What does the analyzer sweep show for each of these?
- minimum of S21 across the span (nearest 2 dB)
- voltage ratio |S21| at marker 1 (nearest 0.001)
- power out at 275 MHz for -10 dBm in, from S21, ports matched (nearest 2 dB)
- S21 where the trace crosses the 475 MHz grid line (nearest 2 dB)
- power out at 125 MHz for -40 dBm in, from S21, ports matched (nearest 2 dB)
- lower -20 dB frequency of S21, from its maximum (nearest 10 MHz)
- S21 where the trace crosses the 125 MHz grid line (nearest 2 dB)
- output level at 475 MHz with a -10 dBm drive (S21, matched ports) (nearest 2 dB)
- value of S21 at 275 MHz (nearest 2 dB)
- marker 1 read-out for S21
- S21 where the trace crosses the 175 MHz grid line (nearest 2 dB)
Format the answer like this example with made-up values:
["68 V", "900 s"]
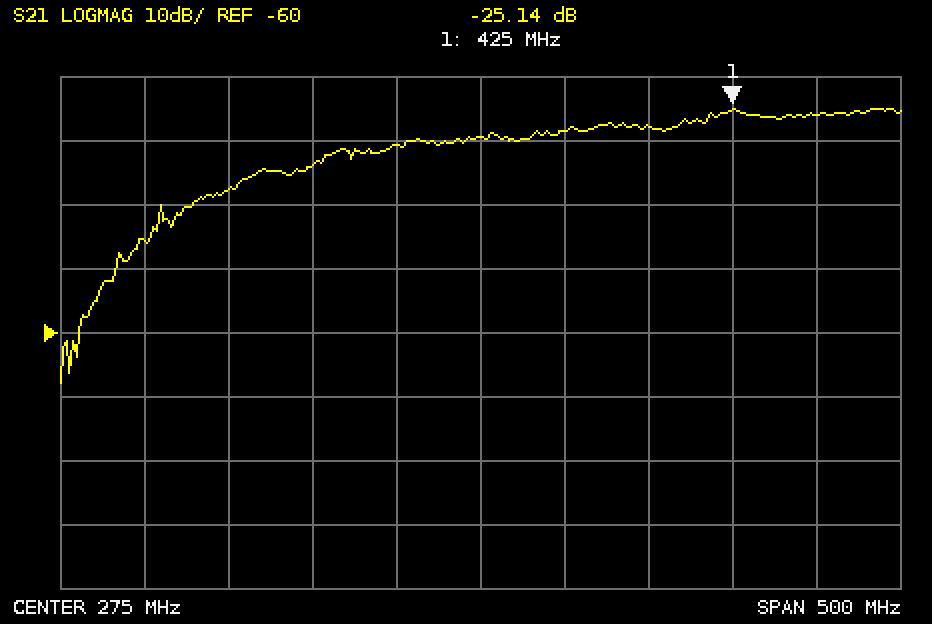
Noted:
["-68 dB", "0.055", "-40 dBm", "-26 dB", "-78 dBm", "80 MHz", "-38 dB", "-36 dBm", "-30 dB", "-25.14 dB", "-34 dB"]
